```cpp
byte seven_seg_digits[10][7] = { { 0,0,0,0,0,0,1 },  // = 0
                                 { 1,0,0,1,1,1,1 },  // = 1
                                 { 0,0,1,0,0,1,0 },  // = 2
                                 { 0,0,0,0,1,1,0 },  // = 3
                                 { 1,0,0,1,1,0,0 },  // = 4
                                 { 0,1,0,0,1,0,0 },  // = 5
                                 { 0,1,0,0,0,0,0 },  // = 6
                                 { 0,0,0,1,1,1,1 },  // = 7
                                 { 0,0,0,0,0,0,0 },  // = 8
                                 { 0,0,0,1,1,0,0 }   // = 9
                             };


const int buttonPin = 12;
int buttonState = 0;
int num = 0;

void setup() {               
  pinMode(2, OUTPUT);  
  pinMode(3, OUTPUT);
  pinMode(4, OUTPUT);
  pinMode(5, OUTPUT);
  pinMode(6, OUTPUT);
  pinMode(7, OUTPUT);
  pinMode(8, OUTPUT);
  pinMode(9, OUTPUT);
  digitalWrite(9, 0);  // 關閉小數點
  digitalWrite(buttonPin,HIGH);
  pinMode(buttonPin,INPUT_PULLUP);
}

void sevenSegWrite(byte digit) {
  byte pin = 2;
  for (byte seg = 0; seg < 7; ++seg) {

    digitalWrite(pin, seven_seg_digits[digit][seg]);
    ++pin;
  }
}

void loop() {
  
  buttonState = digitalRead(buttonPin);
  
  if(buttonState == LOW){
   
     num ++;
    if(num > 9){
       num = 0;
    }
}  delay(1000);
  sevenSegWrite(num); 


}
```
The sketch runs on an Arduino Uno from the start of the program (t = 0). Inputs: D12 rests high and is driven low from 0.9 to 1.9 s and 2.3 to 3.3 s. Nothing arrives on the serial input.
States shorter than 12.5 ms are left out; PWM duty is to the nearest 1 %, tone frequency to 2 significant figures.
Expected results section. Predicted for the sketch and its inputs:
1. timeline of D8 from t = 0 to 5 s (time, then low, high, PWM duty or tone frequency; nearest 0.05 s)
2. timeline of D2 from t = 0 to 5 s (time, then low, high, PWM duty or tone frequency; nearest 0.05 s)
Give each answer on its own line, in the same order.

0 s low; 1 s high; 4 s low
0 s low; 2 s high; 4 s low
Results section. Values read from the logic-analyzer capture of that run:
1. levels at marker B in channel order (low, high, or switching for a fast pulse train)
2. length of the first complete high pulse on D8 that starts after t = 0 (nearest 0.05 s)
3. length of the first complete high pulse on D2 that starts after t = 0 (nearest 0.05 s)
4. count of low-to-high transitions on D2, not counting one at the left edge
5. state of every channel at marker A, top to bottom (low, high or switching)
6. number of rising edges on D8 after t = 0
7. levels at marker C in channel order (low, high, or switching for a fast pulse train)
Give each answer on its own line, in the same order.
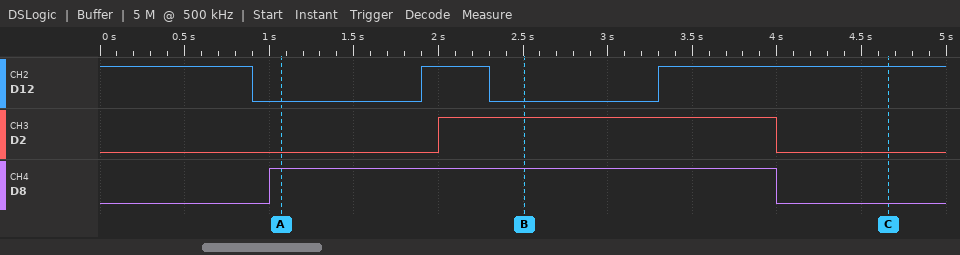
D12 low, D2 high, D8 high
3.00 s
2.00 s
1
D12 low, D2 low, D8 high
1
D12 high, D2 low, D8 low
